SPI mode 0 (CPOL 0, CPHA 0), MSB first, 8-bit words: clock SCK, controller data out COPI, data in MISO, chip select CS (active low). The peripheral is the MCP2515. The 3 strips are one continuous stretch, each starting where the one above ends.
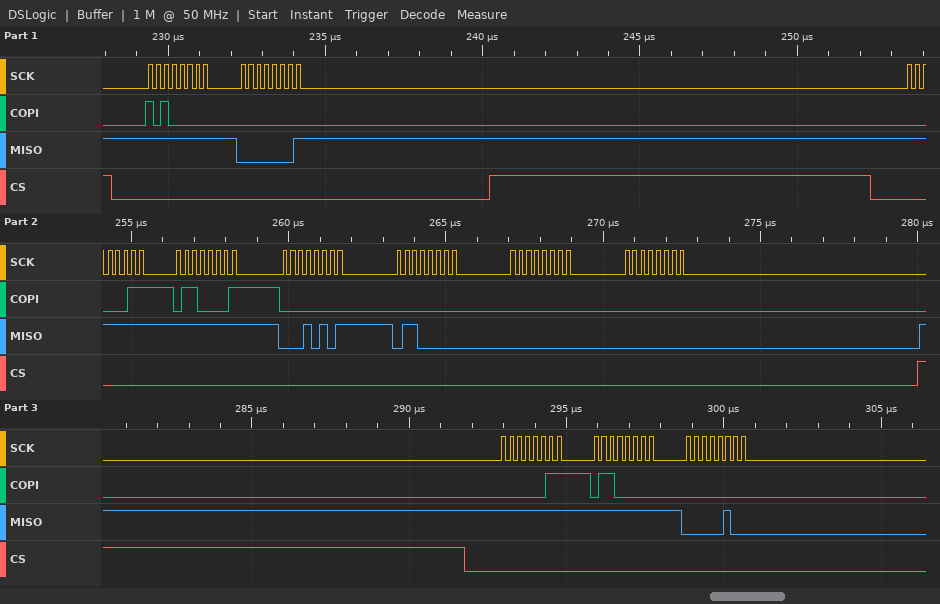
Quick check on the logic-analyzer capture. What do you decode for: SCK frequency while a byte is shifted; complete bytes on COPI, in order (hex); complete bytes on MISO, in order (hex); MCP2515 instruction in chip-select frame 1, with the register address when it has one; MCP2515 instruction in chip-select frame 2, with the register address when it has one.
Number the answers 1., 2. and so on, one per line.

1. 4 MHz
2. A0 00 03 61 00 00 00 00 03 60 00
3. FF 01 FF FF 15 60 00 00 FF FF 04
4. READ STATUS
5. READ 0x61
